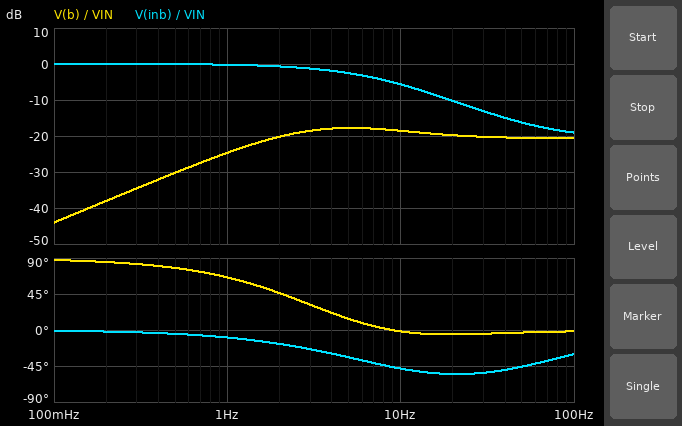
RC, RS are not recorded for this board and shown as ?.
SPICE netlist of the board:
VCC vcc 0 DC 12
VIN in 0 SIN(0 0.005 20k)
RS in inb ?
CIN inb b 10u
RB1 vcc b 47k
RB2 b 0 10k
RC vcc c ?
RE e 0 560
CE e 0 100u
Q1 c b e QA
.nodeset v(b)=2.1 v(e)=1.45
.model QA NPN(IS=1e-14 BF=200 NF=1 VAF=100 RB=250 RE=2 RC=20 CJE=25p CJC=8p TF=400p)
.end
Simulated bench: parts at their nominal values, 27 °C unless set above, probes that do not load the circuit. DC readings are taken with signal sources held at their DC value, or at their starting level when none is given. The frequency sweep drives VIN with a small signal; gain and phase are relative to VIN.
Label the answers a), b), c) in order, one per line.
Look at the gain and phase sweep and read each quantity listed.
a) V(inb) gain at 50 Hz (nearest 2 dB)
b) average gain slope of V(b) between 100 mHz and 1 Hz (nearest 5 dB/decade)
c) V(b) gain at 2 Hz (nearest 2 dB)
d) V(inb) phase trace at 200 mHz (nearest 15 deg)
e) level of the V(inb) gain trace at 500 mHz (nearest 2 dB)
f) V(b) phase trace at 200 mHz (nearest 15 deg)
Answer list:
a) -16 dB
b) 20 dB/decade
c) -20 dB
d) 0 deg
e) 0 dB
f) 90 deg
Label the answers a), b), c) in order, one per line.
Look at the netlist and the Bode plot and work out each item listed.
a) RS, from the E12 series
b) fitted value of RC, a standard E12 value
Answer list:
a) 2.7 kΩ
b) 4.7 kΩ
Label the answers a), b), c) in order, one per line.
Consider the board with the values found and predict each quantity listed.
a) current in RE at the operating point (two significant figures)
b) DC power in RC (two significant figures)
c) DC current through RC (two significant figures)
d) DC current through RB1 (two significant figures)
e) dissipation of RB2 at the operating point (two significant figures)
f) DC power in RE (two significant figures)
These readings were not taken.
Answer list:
a) 2.3 mA
b) 24 mW
c) 2.2 mA
d) 210 µA
e) 380 µW
f) 2.9 mW
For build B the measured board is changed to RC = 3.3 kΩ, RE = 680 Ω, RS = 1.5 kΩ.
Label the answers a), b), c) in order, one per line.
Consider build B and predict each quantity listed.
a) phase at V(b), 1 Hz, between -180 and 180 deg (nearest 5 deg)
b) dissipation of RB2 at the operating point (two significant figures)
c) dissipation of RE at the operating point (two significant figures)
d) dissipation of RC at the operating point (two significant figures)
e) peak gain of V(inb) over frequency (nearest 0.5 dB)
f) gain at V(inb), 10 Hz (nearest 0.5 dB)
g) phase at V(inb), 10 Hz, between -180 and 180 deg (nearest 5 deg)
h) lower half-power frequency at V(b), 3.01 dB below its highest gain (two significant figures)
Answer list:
a) 60 deg
b) 410 µW
c) 2.7 mW
d) 13 mW
e) 0 dB
f) -1.5 dB
g) -5 deg
h) 1.6 Hz
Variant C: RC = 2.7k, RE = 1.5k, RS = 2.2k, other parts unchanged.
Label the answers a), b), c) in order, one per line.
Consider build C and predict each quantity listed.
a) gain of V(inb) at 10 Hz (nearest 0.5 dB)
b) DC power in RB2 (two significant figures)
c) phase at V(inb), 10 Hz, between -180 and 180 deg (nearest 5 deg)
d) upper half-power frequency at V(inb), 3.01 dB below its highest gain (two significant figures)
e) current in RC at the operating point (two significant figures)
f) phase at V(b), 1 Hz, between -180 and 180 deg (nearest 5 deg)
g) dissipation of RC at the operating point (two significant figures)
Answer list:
a) -2.0 dB
b) 430 µW
c) -5 deg
d) 48 Hz
e) 940 µA
f) 55 deg
g) 2.4 mW
